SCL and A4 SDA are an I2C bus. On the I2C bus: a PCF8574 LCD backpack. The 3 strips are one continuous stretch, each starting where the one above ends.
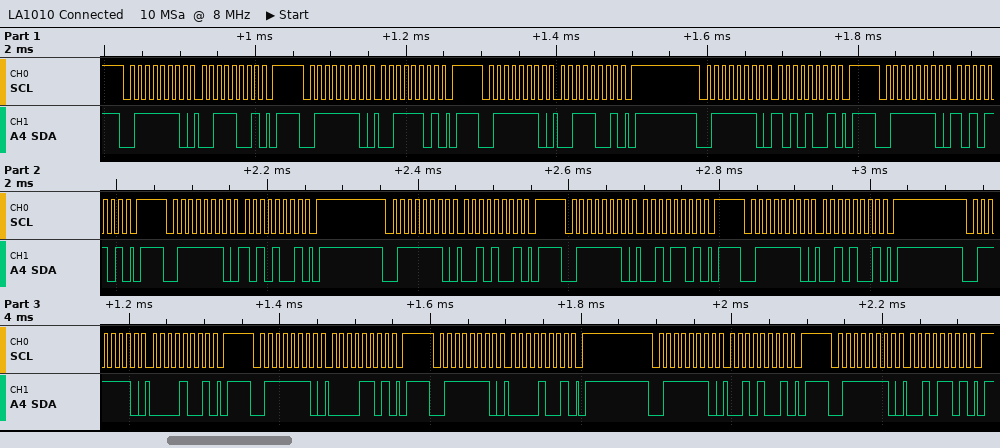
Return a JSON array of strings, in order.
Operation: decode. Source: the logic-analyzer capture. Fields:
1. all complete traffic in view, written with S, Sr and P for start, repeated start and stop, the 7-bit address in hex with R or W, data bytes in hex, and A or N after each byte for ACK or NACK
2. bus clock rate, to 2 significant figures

["S 3FW A 39 A P S 3FW A 3D A P S 3FW A 39 A P S 3FW A A9 A P S 3FW A AD A P S 3FW A A9 A P S 3FW A 29 A P S 3FW A 2D A P S 3FW A 29 A P S 3FW A 09 A P S 3FW A 0D A P S 3FW A 09 A P S 3FW A 29 A P S 3FW A 2D A P", "100 kHz"]
